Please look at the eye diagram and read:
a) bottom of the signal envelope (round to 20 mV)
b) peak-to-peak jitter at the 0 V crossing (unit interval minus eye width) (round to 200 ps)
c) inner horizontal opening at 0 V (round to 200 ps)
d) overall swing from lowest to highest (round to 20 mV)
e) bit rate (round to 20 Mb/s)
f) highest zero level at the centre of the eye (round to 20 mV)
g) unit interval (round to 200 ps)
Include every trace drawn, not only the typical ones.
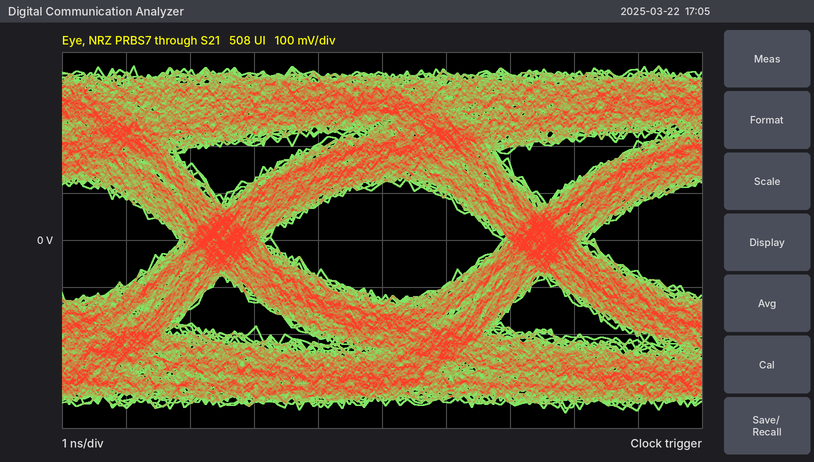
-360 mV
1.4 ns
3.6 ns
740 mV
200 Mb/s
-120 mV
5.0 ns
